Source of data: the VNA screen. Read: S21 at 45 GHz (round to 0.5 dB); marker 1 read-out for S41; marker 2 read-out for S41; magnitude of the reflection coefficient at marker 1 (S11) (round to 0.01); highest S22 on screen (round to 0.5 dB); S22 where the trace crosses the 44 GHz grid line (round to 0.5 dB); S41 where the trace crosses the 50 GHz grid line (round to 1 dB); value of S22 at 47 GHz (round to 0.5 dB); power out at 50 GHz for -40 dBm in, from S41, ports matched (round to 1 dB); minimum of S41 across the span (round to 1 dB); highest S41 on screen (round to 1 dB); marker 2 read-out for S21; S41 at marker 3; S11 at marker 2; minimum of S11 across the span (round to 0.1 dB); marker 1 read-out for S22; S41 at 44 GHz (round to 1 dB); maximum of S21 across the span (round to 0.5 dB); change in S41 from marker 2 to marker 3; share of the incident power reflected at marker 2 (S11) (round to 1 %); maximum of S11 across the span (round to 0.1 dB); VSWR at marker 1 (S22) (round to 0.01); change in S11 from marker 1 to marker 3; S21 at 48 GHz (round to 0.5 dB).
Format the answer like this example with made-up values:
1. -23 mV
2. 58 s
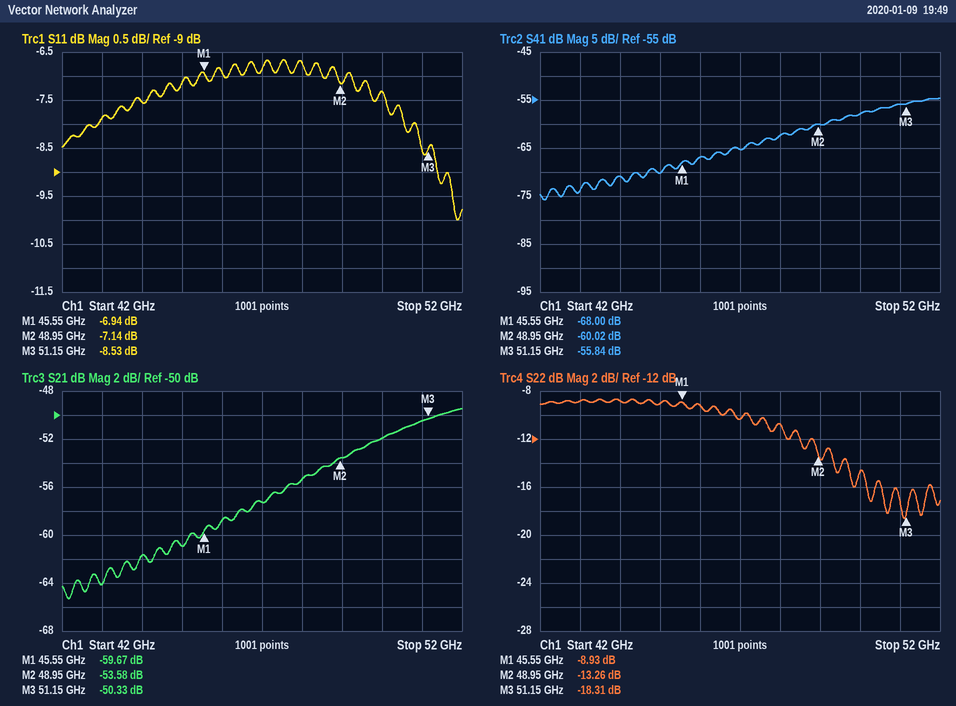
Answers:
1. -61.0 dB
2. -68.00 dB
3. -60.02 dB
4. 0.45
5. -8.5 dB
6. -9.0 dB
7. -58 dB
8. -10.5 dB
9. -98 dBm
10. -76 dB
11. -55 dB
12. -53.58 dB
13. -55.84 dB
14. -7.14 dB
15. -10.0 dB
16. -8.93 dB
17. -71 dB
18. -49.5 dB
19. 4.18 dB
20. 19 %
21. -6.7 dB
22. 2.11
23. -1.59 dB
24. -55.5 dB
